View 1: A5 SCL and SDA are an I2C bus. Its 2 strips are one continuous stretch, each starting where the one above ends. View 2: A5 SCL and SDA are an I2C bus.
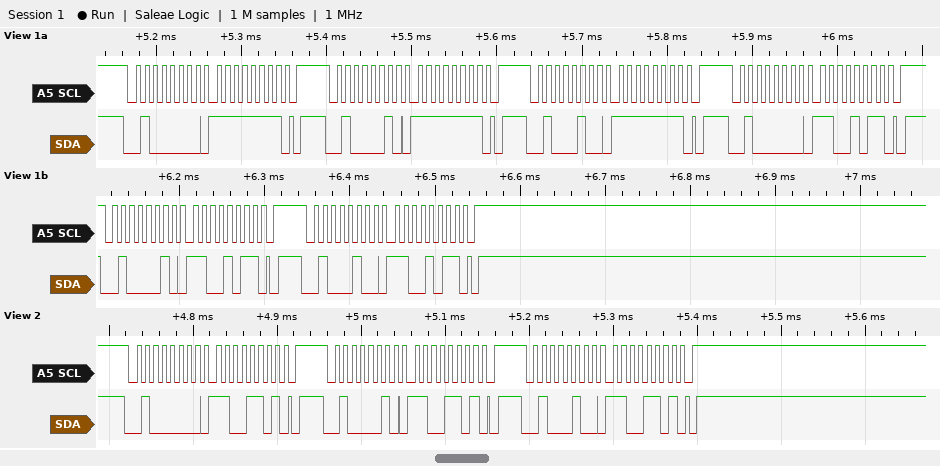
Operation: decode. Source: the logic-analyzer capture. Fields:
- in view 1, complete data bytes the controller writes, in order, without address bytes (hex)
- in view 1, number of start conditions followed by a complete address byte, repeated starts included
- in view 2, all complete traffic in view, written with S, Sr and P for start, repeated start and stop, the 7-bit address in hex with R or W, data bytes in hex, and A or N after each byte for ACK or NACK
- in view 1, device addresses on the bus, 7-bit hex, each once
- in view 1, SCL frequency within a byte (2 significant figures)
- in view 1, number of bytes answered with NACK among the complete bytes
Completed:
FF FF FF CB CB CB
6
S 20W A CD A P S 21W A CD A P S 22W A CD A P
0x20 0x21 0x22
100 kHz
0
